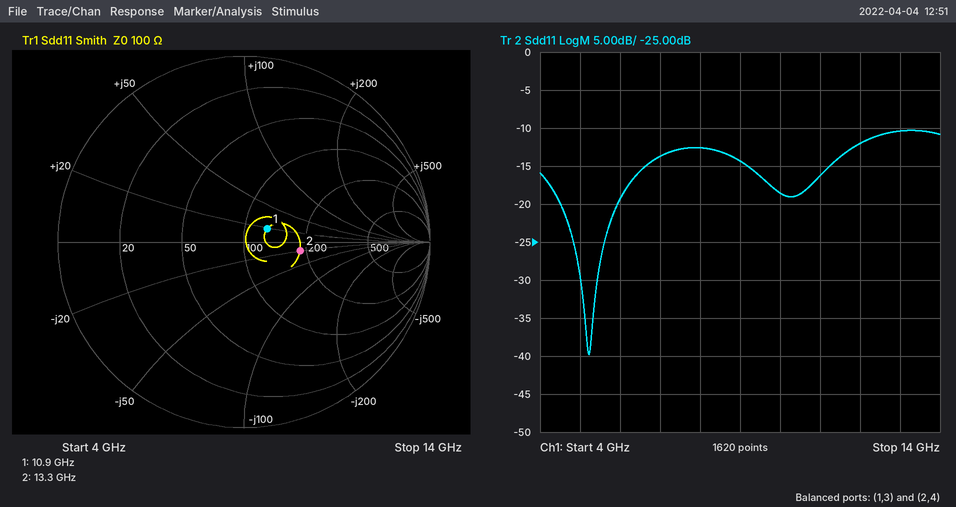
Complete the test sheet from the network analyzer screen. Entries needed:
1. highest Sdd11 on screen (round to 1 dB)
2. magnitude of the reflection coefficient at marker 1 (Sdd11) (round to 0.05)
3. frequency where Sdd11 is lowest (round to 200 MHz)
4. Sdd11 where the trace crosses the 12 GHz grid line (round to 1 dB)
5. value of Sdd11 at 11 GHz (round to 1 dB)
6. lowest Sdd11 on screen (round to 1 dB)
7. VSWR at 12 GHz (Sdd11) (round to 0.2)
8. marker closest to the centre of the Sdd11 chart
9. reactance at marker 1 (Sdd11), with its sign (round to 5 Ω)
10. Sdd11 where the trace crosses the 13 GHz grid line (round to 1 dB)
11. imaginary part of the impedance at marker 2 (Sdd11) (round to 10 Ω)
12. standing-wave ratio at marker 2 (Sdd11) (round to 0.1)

-10 dB
0.15
5.2 GHz
-12 dB
-16 dB
-40 dB
1.6
marker 1
+20 Ω
-10 dB
-20 Ω
1.9
